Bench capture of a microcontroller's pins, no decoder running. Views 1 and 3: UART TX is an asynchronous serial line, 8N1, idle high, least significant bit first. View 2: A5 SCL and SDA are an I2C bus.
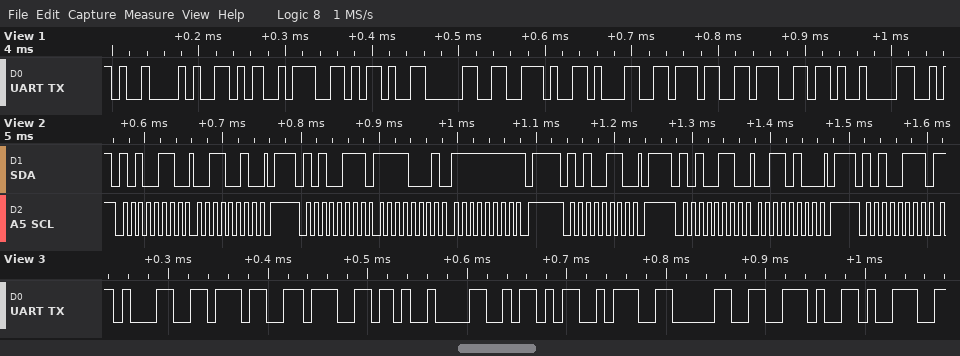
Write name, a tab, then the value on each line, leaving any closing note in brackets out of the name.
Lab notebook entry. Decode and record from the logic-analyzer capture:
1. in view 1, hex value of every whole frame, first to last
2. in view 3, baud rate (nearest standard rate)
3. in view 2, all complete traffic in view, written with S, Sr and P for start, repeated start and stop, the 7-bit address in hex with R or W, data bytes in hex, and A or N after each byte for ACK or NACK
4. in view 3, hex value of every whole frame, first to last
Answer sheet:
in view 1, hex value of every whole frame, first to last	09 59 3A 2D 30 2E 31 37 67 09
in view 3, baud rate	115200 baud
in view 2, all complete traffic in view, written with S, Sr and P for start, repeated start and stop, the 7-bit address in hex with R or W, data bytes in hex, and A or N after each byte for ACK or NACK	S 53W A 32 A P S 53R A F1 A FF N P S 53W A P S 53W A 34 A P S 53R A
in view 3, hex value of every whole frame, first to last	31 37 67 09 5A 3A 30 2E 39
